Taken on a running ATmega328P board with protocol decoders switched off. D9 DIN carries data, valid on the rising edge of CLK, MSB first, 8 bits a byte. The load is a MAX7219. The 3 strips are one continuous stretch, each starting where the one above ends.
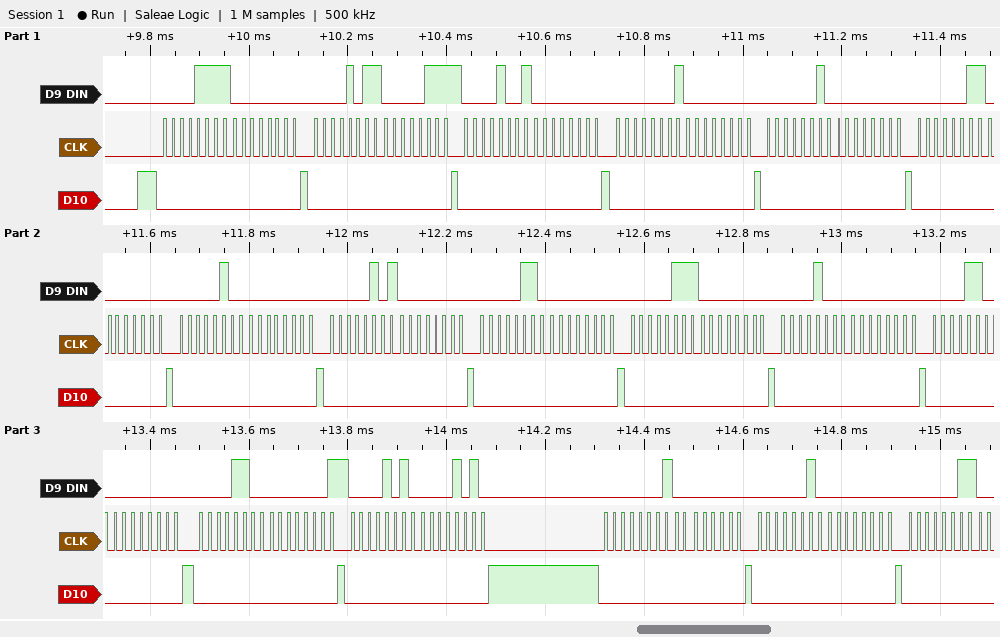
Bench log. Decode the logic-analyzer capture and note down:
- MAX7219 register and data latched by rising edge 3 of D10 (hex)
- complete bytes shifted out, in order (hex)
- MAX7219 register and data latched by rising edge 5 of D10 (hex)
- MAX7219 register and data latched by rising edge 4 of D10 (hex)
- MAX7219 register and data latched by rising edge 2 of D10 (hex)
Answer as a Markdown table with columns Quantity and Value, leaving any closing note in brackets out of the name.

| Quantity | Value |
|---|---|
| MAX7219 register and data latched by rising edge 3 of D10 | register 0xB, data 0x07 |
| complete bytes shifted out, in order | 0x0F 0x00 0x0B 0x07 0x09 0x00 0x01 0x00 0x02 0x00 0x03 0x00 0x04 0x00 0x05 0x00 0x06 0x00 0x07 0x00 0x08 0x00 0x0C 0x00 0x0C 0x01 0x0A 0x0A 0x01 0x00 0x02 0x00 0x03 |
| MAX7219 register and data latched by rising edge 5 of D10 | register 0x1, data 0x00 |
| MAX7219 register and data latched by rising edge 4 of D10 | register 0x9, data 0x00 |
| MAX7219 register and data latched by rising edge 2 of D10 | register 0xF, data 0x00 |
